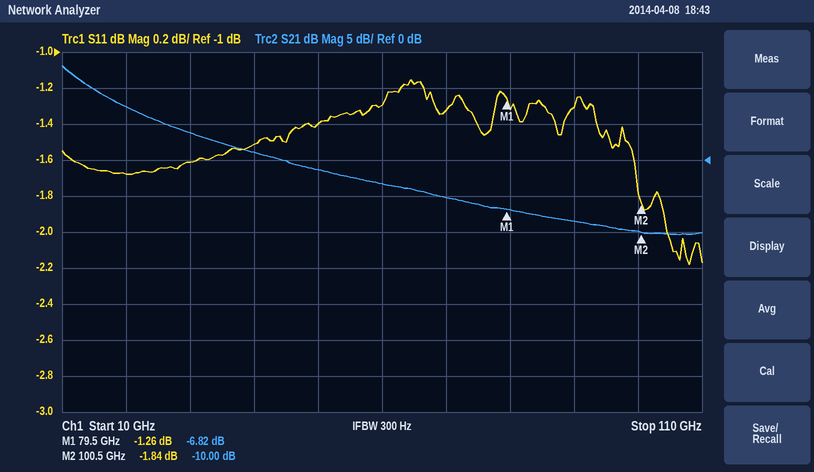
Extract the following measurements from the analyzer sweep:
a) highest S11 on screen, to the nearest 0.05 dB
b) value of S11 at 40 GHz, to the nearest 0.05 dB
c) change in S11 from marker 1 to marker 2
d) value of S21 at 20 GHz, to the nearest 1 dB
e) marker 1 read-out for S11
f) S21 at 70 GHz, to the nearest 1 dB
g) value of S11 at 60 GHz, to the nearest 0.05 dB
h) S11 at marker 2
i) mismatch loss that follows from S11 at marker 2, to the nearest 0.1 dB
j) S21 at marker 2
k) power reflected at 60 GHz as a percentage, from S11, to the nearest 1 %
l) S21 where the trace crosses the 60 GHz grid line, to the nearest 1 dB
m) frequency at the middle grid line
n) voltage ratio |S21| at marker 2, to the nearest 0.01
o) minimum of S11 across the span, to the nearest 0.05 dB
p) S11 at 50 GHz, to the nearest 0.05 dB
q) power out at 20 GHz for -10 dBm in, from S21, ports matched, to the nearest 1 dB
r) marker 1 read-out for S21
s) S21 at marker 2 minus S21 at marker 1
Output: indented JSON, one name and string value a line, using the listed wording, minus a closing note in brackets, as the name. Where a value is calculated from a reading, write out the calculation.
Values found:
{
  "highest S11 on screen, to the nearest 0.05 dB": "-1.15 dB",
  "value of S11 at 40 GHz, to the nearest 0.05 dB": "-1.50 dB",
  "change in S11 from marker 1 to marker 2": "-1.84 − (-1.26) = -0.58 dB",
  "value of S21 at 20 GHz, to the nearest 1 dB": "7 dB",
  "marker 1 read-out for S11": "-1.26 dB",
  "S21 at 70 GHz, to the nearest 1 dB": "-5 dB",
  "value of S11 at 60 GHz, to the nearest 0.05 dB": "-1.30 dB",
  "S11 at marker 2": "-1.84 dB",
  "mismatch loss that follows from S11 at marker 2, to the nearest 0.1 dB": "−10 log10(1 − 10^(-1.84/10)) ≈ 4.6 dB",
  "S21 at marker 2": "-10.00 dB",
  "power reflected at 60 GHz as a percentage, from S11, to the nearest 1 %": "10^(-1.3/10) ≈ 74 %",
  "S21 where the trace crosses the 60 GHz grid line, to the nearest 1 dB": "-3 dB",
  "frequency at the middle grid line": "60 GHz",
  "voltage ratio |S21| at marker 2, to the nearest 0.01": "10^(-10/20) ≈ 0.32",
  "minimum of S11 across the span, to the nearest 0.05 dB": "-2.20 dB",
  "S11 at 50 GHz, to the nearest 0.05 dB": "-1.40 dB",
  "power out at 20 GHz for -10 dBm in, from S21, ports matched, to the nearest 1 dB": "-10 dBm + (7 dB) = -3 dBm",
  "marker 1 read-out for S21": "-6.82 dB",
  "S21 at marker 2 minus S21 at marker 1": "-10 − (-6.82) = -3.18 dB"
}
